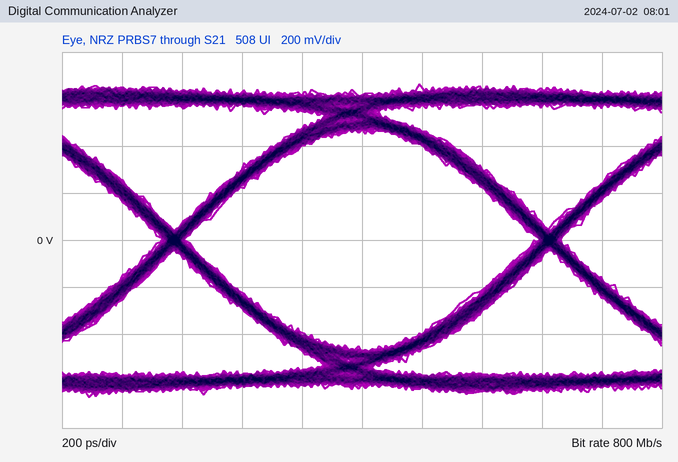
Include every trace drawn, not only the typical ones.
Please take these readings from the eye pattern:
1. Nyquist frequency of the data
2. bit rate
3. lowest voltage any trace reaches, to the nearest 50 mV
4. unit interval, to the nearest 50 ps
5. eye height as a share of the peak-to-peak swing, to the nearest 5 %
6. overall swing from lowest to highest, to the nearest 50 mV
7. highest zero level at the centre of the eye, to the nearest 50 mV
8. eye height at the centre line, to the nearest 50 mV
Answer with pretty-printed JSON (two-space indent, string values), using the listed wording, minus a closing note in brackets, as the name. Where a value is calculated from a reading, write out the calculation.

{
  "Nyquist frequency of the data": "400 MHz",
  "bit rate": "800 Mb/s",
  "lowest voltage any trace reaches, to the nearest 50 mV": "-650 mV",
  "unit interval, to the nearest 50 ps": "1.25 ns",
  "eye height as a share of the peak-to-peak swing, to the nearest 5 %": "950 mV / 1.35 V ≈ 70 %",
  "overall swing from lowest to highest, to the nearest 50 mV": "1.35 V",
  "highest zero level at the centre of the eye, to the nearest 50 mV": "-450 mV",
  "eye height at the centre line, to the nearest 50 mV": "950 mV"
}
